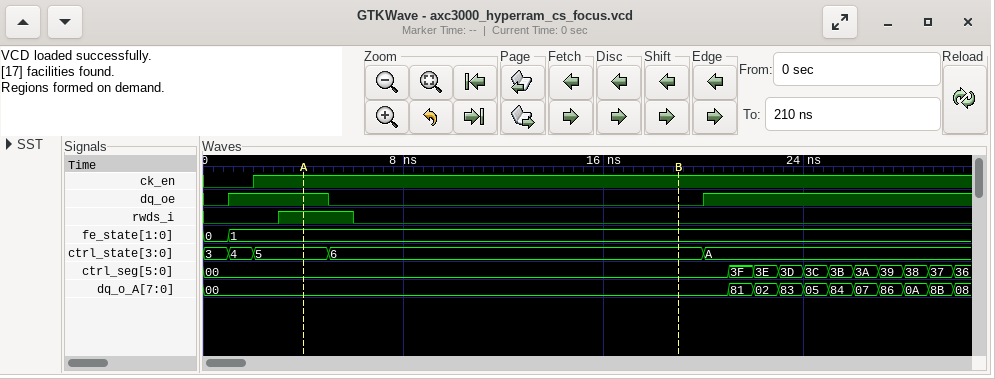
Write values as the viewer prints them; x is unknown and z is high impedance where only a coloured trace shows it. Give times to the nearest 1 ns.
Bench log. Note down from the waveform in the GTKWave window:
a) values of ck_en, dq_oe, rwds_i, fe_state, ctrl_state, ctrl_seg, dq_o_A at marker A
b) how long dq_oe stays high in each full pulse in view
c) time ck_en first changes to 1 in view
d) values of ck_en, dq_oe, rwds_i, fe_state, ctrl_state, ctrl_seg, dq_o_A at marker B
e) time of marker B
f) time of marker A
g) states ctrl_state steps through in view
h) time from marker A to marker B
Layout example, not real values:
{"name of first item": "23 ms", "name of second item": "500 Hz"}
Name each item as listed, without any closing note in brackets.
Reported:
{"values of ck_en, dq_oe, rwds_i, fe_state, ctrl_state, ctrl_seg, dq_o_A at marker A": "ck_en=1, dq_oe=1, rwds_i=1, fe_state=1, ctrl_state=5, ctrl_seg=00, dq_o_A=00", "how long dq_oe stays high in each full pulse in view": "4 ns", "time ck_en first changes to 1 in view": "2 ns", "values of ck_en, dq_oe, rwds_i, fe_state, ctrl_state, ctrl_seg, dq_o_A at marker B": "ck_en=1, dq_oe=0, rwds_i=0, fe_state=1, ctrl_state=6, ctrl_seg=00, dq_o_A=00", "time of marker B": "19 ns", "time of marker A": "4 ns", "states ctrl_state steps through in view": "3, 4, 5, 6, A", "time from marker A to marker B": "15 ns"}
